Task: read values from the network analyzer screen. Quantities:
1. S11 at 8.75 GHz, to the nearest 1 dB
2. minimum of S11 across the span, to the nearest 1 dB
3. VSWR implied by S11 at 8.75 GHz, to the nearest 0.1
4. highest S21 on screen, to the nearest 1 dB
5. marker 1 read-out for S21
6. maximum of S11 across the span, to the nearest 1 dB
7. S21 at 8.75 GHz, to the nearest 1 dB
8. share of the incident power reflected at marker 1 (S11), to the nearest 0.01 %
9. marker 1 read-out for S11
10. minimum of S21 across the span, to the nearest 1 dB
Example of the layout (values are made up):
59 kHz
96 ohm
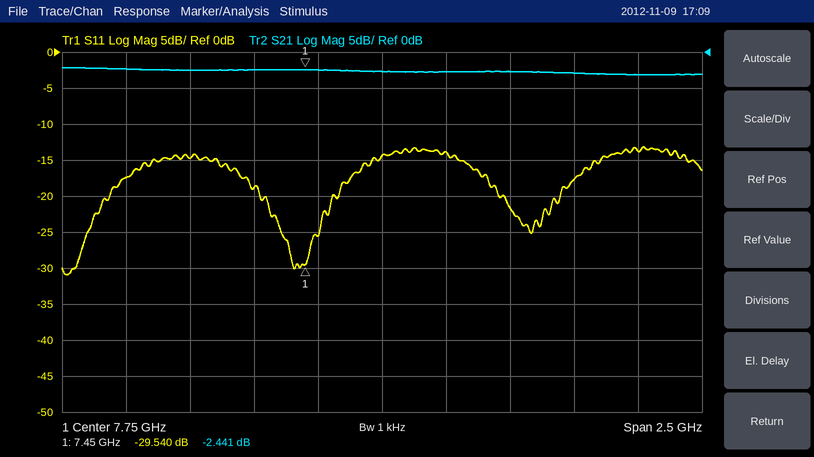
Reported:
-14 dB
-31 dB
1.5
-2 dB
-2.441 dB
-13 dB
-3 dB
0.11 %
-29.540 dB
-3 dB
